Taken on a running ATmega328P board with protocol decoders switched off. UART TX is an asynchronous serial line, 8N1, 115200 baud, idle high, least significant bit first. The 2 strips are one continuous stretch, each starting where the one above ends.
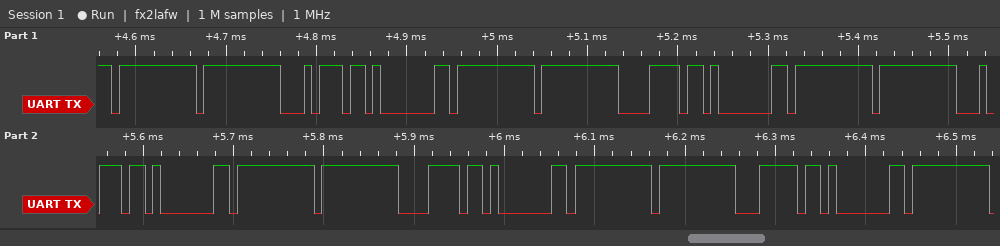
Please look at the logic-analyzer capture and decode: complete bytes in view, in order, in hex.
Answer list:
0xFF 0xFF 0x74 0x01 0xFF 0xFF 0x78 0x01 0xFF 0xFF 0x74 0x01 0xFF 0xFF 0x78 0x01 0xFF 0xFF 0x7C 0x01 0xFF
